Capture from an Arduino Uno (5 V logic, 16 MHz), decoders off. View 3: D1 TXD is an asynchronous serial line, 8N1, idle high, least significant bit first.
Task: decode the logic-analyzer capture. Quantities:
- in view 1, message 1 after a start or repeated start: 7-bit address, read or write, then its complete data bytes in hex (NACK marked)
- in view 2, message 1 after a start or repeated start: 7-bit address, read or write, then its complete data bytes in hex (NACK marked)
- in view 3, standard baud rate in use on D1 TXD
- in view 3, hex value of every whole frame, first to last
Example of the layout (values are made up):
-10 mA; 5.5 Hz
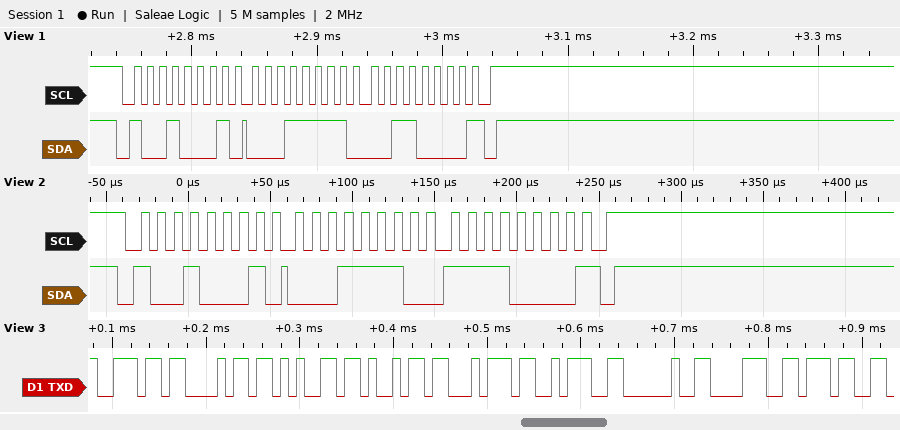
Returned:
0x48 read: 1F 30 NACK; 0x48 read: 1E F0 NACK; 115200 baud; 6E 68 65 69 74 3A 20 38 37
